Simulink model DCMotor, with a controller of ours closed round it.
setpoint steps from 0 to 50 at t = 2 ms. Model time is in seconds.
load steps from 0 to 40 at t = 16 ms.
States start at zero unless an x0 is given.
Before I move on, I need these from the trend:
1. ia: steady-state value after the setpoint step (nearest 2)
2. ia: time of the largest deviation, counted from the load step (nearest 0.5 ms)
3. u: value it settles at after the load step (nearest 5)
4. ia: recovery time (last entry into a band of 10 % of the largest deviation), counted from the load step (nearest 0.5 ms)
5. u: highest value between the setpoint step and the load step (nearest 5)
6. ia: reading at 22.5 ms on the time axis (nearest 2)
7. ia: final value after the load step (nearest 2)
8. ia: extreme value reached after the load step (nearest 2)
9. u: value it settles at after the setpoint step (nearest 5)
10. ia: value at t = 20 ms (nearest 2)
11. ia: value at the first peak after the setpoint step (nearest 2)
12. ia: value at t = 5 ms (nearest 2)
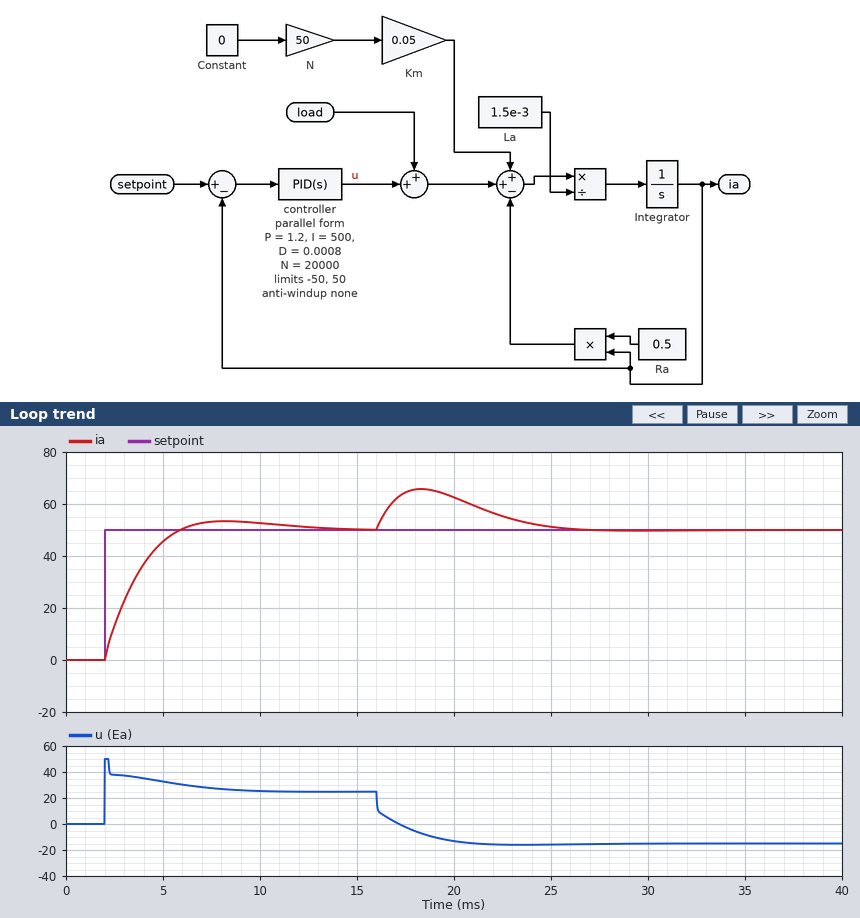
50
2.5 ms
-15
8.5 ms
50
56
50
66
25
62
54
46
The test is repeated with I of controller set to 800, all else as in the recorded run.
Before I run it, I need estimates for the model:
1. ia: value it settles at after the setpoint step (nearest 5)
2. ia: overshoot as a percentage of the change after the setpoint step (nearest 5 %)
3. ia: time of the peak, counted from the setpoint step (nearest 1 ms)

50
15 %
5 ms
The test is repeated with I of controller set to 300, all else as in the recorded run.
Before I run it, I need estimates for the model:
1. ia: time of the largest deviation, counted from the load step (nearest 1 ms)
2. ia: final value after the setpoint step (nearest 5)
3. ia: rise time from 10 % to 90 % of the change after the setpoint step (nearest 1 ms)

3 ms
50
4 ms
